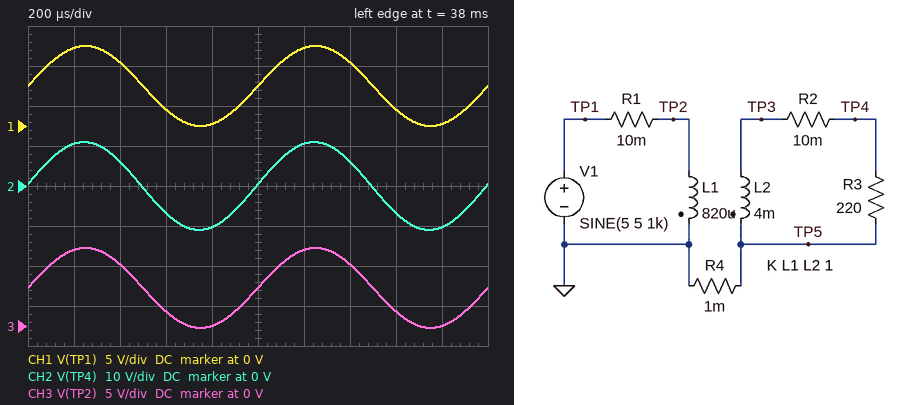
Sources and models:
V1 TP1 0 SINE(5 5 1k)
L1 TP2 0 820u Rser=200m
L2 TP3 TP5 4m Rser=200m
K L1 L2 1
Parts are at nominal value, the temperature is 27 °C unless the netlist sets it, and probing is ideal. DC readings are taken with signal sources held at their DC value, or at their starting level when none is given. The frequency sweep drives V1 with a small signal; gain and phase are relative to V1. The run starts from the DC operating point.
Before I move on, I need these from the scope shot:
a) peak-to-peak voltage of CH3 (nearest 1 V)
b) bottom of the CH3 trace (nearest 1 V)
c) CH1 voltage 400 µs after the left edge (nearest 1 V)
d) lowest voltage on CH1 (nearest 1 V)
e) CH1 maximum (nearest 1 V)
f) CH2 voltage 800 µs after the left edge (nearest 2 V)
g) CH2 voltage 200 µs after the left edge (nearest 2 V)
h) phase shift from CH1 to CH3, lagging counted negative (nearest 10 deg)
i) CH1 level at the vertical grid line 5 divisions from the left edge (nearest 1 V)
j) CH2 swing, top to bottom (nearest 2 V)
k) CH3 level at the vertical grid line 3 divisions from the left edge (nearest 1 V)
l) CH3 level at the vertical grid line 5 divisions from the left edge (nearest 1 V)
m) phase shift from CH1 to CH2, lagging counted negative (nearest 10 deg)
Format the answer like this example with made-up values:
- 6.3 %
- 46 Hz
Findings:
- 10 V
- 0 V
- 8 V
- 0 V
- 10 V
- -10 V
- 10 V
- 0 deg
- 5 V
- 22 V
- 2 V
- 5 V
- 0 deg
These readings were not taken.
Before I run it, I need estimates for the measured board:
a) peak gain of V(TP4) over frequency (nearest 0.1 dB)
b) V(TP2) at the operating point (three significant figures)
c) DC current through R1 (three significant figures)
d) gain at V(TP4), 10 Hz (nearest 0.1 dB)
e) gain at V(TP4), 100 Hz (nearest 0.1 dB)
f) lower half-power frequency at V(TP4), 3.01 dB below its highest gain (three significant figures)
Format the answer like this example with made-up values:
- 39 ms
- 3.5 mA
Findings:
- 6.8 dB
- 4.76 V
- 23.8 A
- -5.6 dB
- 6.2 dB
- 40.6 Hz
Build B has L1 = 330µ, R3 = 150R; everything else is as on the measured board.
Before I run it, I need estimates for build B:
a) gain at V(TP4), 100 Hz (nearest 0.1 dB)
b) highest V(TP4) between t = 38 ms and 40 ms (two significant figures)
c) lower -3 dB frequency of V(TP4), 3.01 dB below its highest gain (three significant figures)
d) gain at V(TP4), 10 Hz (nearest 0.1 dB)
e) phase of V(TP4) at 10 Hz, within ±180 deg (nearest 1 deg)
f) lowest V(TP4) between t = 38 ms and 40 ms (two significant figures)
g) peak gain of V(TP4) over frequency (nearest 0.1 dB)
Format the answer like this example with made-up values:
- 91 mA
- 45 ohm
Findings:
- 7.7 dB
- 17 V
- 99.6 Hz
- -9.3 dB
- 84 deg
- -17 V
- 10.7 dB
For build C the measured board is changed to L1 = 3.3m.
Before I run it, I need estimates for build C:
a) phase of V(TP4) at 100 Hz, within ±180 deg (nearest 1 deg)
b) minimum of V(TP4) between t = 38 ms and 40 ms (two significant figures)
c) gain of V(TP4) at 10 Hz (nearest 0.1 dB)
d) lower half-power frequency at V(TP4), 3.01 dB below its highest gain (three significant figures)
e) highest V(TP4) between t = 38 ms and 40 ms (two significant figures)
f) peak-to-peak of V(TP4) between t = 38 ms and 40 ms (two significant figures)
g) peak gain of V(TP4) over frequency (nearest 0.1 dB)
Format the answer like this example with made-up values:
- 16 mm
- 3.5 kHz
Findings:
- 6 deg
- -5.5 V
- -2.2 dB
- 10.1 Hz
- 5.5 V
- 11 V
- 0.8 dB
